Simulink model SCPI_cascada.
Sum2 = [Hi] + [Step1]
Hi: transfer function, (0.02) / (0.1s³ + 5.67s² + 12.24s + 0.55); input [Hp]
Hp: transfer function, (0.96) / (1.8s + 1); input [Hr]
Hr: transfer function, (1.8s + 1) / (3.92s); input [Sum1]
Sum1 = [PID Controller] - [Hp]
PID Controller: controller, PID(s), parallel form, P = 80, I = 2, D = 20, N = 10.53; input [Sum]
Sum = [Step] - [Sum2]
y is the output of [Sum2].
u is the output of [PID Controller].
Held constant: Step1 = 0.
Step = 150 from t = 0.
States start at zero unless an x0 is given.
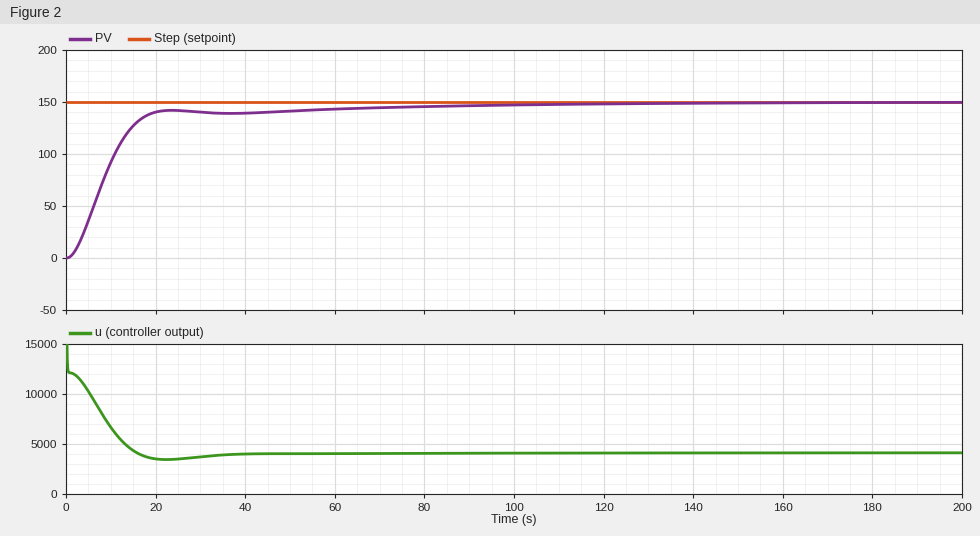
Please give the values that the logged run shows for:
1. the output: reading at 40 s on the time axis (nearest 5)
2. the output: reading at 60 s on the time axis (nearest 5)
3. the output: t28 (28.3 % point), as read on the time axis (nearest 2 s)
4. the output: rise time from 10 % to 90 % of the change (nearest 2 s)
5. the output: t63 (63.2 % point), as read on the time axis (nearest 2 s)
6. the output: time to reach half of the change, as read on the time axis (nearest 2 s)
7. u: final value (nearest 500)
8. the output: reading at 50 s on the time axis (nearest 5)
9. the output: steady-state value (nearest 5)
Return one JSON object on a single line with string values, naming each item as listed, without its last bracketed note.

{"the output: reading at 40 s on the time axis": "140", "the output: reading at 60 s on the time axis": "145", "the output: t28 (28.3 % point), as read on the time axis": "6 s", "the output: rise time from 10 % to 90 % of the change": "14 s", "the output: t63 (63.2 % point), as read on the time axis": "10 s", "the output: time to reach half of the change, as read on the time axis": "8 s", "u: final value": "4000", "the output: reading at 50 s on the time axis": "140", "the output: steady-state value": "150"}
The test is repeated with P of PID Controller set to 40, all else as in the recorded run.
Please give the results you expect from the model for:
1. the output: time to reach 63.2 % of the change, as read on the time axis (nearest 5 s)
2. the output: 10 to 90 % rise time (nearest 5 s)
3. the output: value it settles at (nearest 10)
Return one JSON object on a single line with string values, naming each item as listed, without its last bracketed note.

{"the output: time to reach 63.2 % of the change, as read on the time axis": "15 s", "the output: 10 to 90 % rise time": "25 s", "the output: value it settles at": "150"}
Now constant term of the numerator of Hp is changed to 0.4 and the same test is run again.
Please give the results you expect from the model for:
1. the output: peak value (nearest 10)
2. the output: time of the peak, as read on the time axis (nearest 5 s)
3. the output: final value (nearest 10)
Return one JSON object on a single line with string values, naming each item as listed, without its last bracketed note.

{"the output: peak value": "160", "the output: time of the peak, as read on the time axis": "30 s", "the output: final value": "150"}
